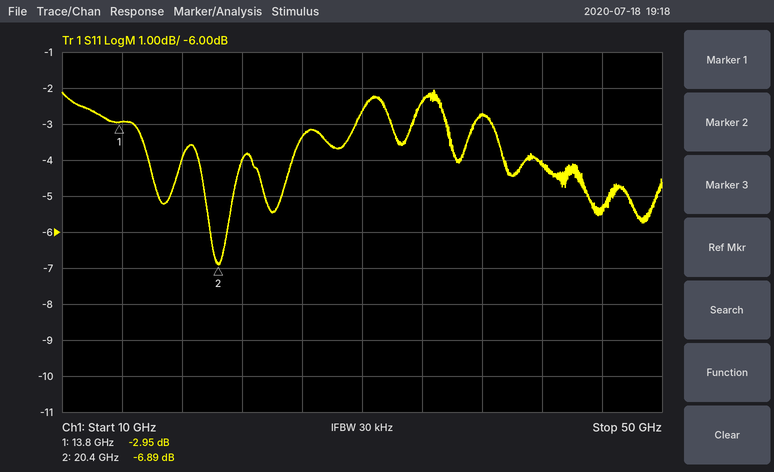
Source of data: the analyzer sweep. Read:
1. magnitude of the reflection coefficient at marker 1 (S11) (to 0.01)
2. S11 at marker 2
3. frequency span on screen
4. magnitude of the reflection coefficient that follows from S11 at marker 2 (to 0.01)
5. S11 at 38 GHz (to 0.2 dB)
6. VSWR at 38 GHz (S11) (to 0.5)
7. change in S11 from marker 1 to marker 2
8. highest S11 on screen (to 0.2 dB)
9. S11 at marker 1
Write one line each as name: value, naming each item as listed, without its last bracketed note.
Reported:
magnitude of the reflection coefficient at marker 1 (S11): 0.71
S11 at marker 2: -6.89 dB
frequency span on screen: 40 GHz
magnitude of the reflection coefficient that follows from S11 at marker 2: 0.45
S11 at 38 GHz: -2.8 dB
VSWR at 38 GHz (S11): 6.5
change in S11 from marker 1 to marker 2: -3.94 dB
highest S11 on screen: -2.0 dB
S11 at marker 1: -2.95 dB
